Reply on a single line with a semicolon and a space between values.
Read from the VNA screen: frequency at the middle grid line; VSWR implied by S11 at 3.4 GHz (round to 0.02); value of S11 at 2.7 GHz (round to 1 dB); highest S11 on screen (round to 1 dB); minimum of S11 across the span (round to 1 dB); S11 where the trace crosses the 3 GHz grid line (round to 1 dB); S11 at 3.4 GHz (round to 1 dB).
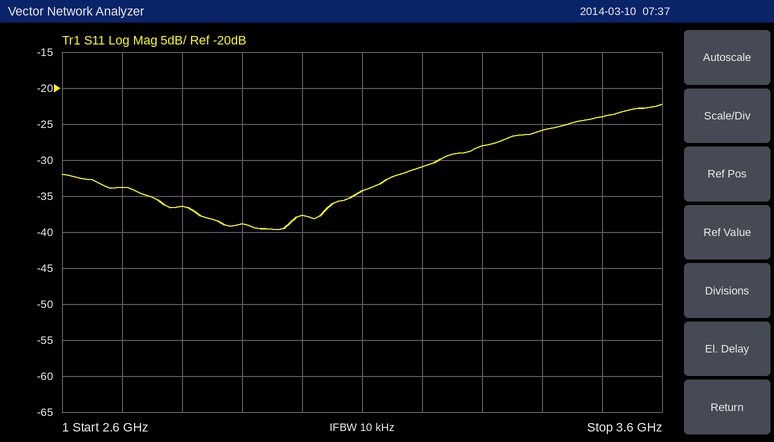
3.1 GHz; 1.10; -34 dB; -22 dB; -40 dB; -38 dB; -26 dB
